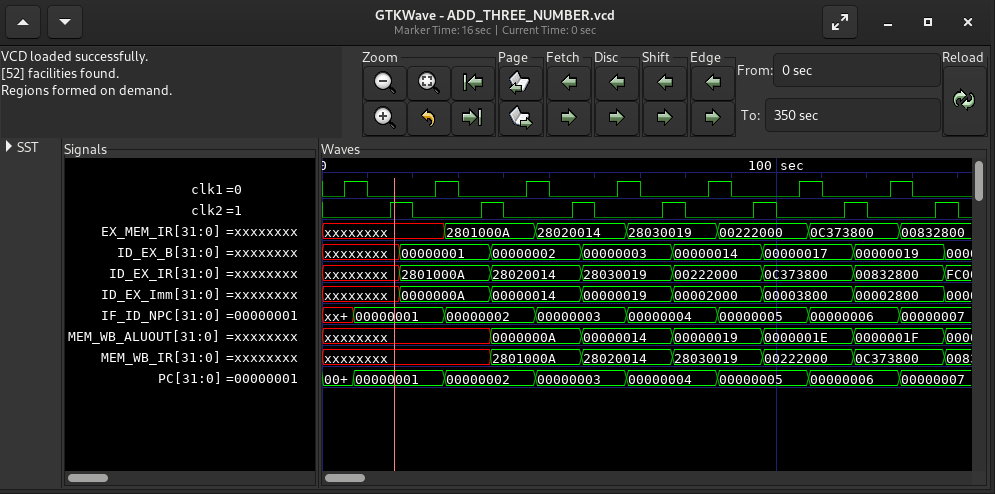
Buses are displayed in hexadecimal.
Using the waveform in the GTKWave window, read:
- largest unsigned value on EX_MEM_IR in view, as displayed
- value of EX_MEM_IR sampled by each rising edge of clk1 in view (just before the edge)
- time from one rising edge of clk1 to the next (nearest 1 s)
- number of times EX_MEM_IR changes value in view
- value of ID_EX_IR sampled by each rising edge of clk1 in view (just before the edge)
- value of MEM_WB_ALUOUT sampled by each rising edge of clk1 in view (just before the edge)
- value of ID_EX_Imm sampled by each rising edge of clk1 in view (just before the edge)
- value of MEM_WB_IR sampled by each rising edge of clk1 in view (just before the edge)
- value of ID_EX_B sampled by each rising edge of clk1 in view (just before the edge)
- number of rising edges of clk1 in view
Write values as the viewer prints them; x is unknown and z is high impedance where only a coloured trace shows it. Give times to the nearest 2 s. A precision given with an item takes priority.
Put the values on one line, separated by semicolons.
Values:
28030019; xxxxxxxx, xxxxxxxx, 2801000A, 28020014, 28030019, 00222000, 0C373800; 20 s; 6; xxxxxxxx, 2801000A, 28020014, 28030019, 00222000, 0C373800, 00832800; xxxxxxxx, xxxxxxxx, 0000000A, 00000014, 00000019, 0000001E, 0000001F; xxxxxxxx, 0000000A, 00000014, 00000019, 00002000, 00003800, 00002800; xxxxxxxx, xxxxxxxx, 2801000A, 28020014, 28030019, 00222000, 0C373800; xxxxxxxx, 00000001, 00000002, 00000003, 00000014, 00000017, 00000019; 7
